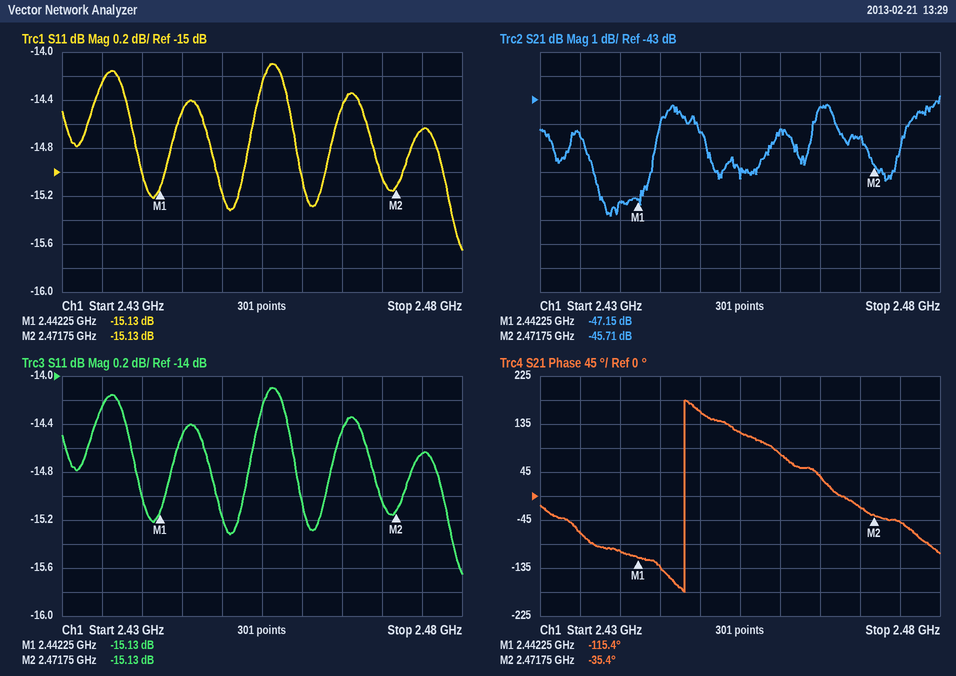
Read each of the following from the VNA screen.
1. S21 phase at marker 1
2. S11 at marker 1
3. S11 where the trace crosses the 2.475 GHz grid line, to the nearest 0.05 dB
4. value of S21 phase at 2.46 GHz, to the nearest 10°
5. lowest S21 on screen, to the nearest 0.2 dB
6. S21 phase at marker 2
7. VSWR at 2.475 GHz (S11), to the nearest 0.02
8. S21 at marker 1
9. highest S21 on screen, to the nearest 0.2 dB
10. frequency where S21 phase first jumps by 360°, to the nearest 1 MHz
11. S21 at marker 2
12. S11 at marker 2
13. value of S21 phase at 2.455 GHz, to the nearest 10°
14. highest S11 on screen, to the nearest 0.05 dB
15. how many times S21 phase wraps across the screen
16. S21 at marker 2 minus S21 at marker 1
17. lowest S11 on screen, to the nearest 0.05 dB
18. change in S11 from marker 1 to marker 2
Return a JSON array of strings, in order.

["-115.4°", "-15.13 dB", "-14.65 dB", "80°", "-47.8 dB", "-35.4°", "1.46", "-47.15 dB", "-42.8 dB", "2.448 GHz", "-45.71 dB", "-15.13 dB", "120°", "-14.10 dB", "1", "1.44 dB", "-15.65 dB", "0.00 dB"]
